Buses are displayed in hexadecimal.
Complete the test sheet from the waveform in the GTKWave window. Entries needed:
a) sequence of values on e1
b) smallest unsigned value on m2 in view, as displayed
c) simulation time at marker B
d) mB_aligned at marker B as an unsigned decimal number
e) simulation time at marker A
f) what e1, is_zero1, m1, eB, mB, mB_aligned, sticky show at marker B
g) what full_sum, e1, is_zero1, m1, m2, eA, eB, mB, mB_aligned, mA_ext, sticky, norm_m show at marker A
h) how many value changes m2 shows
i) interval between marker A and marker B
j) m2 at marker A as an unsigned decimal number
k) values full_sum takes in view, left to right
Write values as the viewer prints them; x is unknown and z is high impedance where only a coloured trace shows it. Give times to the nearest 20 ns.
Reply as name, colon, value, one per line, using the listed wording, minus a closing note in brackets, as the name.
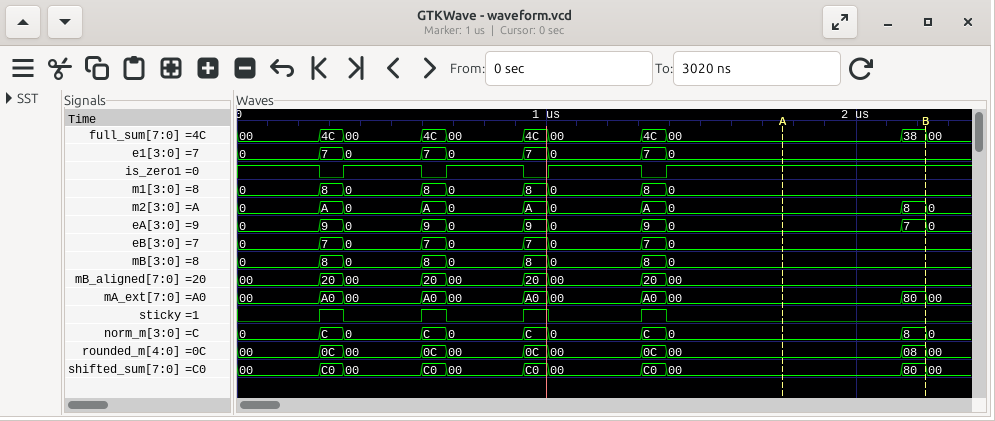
sequence of values on e1: 0, 7, 0, 7, 0, 7, 0, 7, 0
smallest unsigned value on m2 in view, as displayed: 0
simulation time at marker B: 2220 ns
mB_aligned at marker B as an unsigned decimal number: 0
simulation time at marker A: 1760 ns
what e1, is_zero1, m1, eB, mB, mB_aligned, sticky show at marker B: e1=0, is_zero1=1, m1=0, eB=0, mB=0, mB_aligned=00, sticky=0
what full_sum, e1, is_zero1, m1, m2, eA, eB, mB, mB_aligned, mA_ext, sticky, norm_m show at marker A: full_sum=00, e1=0, is_zero1=1, m1=0, m2=0, eA=0, eB=0, mB=0, mB_aligned=00, mA_ext=00, sticky=0, norm_m=0
how many value changes m2 shows: 10
interval between marker A and marker B: 460 ns
m2 at marker A as an unsigned decimal number: 0
values full_sum takes in view, left to right: 00, 4C, 00, 4C, 00, 4C, 00, 4C, 00, 38, 00
